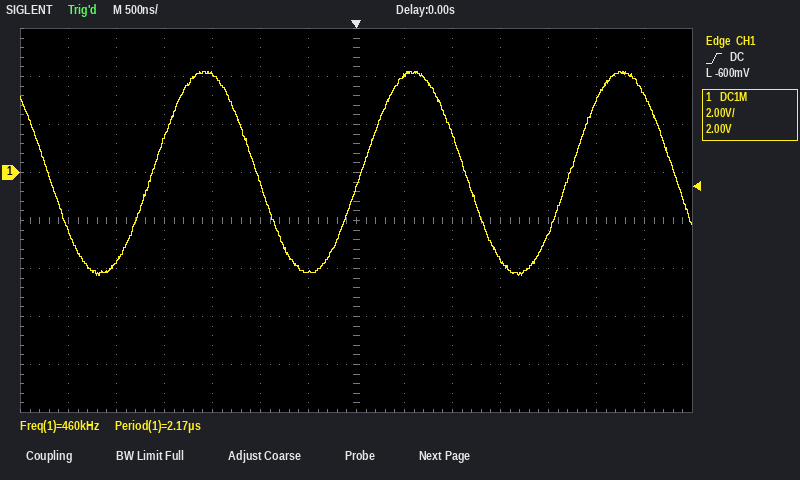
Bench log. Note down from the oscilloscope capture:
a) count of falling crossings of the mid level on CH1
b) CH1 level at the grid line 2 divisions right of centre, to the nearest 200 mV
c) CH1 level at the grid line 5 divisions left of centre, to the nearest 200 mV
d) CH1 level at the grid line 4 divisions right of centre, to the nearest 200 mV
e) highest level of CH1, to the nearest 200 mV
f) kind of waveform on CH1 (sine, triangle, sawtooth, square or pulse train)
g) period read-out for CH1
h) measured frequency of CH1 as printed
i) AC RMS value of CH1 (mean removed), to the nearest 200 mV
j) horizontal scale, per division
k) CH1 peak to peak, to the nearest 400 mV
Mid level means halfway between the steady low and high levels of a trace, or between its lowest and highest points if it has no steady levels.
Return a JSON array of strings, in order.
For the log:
["4", "1.6 V", "-3.8 V", "-2.6 V", "4.2 V", "sine", "2.17 µs", "460 kHz", "3.0 V", "500 ns", "8.4 V"]
